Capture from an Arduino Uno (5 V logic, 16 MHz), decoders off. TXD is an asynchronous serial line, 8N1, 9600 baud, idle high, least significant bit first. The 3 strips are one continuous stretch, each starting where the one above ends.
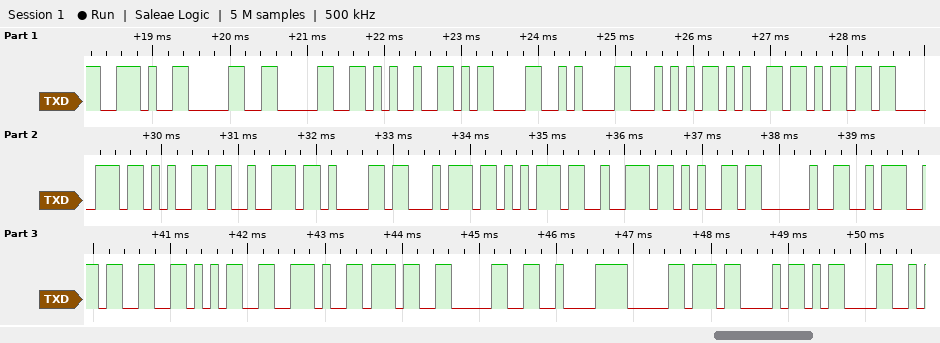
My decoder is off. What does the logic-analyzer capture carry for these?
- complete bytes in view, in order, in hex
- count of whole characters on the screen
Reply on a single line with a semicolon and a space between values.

0x2E 0x30 0x30 0x25 0x0D 0x0A 0x54 0x65 0x6D 0x70 0x65 0x72 0x61 0x74 0x75 0x72 0x65 0x20 0x3A 0x33 0x35 0x2E 0x37 0x30 0xC2 0xB0 0x43 0x0D; 28
